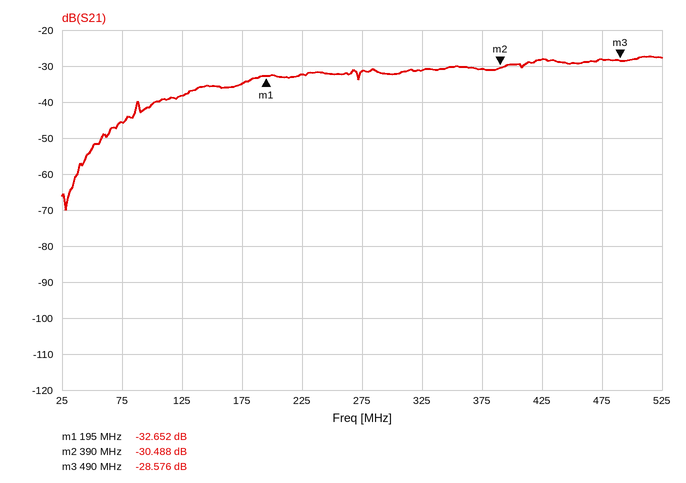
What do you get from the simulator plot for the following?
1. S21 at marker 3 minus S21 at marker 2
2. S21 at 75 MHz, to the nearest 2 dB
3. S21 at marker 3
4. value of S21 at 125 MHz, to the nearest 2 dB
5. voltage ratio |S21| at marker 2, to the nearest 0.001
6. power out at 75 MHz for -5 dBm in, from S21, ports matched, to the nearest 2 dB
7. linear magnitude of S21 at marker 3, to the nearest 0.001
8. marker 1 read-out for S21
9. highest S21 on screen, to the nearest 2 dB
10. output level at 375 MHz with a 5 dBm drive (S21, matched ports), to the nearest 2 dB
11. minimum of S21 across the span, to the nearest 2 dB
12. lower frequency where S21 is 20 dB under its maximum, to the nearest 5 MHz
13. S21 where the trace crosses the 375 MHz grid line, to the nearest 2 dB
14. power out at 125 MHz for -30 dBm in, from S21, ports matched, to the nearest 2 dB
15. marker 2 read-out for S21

1.912 dB
-46 dB
-28.576 dB
-38 dB
0.030
-50 dBm
0.037
-32.652 dB
-28 dB
-26 dBm
-70 dB
65 MHz
-30 dB
-68 dBm
-30.488 dB
